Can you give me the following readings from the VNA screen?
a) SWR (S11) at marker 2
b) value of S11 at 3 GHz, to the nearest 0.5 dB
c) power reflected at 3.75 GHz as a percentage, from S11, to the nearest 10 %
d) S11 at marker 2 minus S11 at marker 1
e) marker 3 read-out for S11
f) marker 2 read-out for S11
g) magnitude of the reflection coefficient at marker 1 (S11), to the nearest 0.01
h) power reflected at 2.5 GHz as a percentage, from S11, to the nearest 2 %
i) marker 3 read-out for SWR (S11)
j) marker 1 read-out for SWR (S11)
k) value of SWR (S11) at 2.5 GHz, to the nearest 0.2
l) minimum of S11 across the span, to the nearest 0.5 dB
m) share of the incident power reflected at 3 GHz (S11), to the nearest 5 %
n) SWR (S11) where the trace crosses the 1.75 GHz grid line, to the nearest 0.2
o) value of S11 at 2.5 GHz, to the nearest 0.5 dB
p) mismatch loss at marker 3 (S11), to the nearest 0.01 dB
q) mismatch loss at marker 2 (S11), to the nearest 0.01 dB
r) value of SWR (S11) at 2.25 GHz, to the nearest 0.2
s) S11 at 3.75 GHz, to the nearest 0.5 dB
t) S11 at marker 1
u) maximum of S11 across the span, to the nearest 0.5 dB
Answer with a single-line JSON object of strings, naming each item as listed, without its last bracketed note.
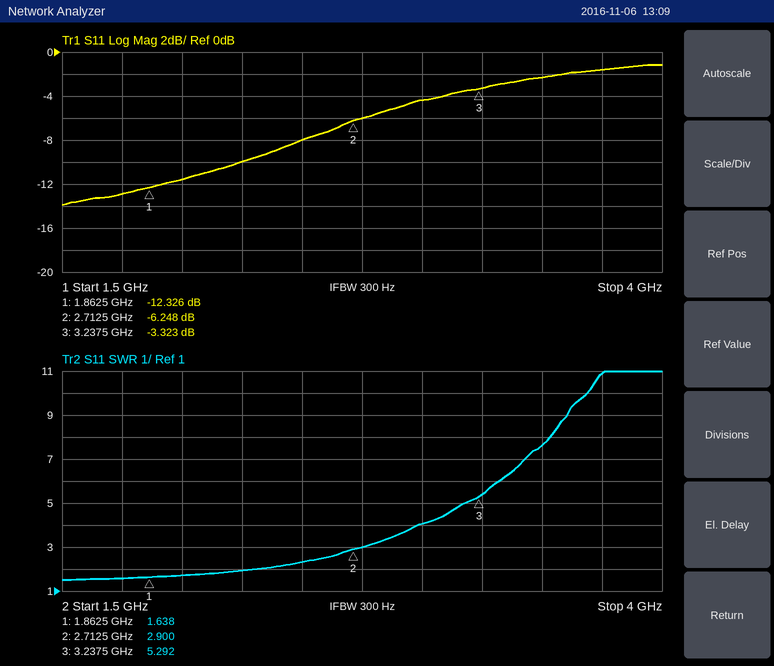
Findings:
{"SWR (S11) at marker 2": "2.900", "value of S11 at 3 GHz, to the nearest 0.5 dB": "-4.5 dB", "power reflected at 3.75 GHz as a percentage, from S11, to the nearest 10 %": "70 %", "S11 at marker 2 minus S11 at marker 1": "6.078 dB", "marker 3 read-out for S11": "-3.323 dB", "marker 2 read-out for S11": "-6.248 dB", "magnitude of the reflection coefficient at marker 1 (S11), to the nearest 0.01": "0.24", "power reflected at 2.5 GHz as a percentage, from S11, to the nearest 2 %": "16 %", "marker 3 read-out for SWR": "5.292", "marker 1 read-out for SWR": "1.638", "value of SWR (S11) at 2.5 GHz, to the nearest 0.2": "2.4", "minimum of S11 across the span, to the nearest 0.5 dB": "-14.0 dB", "share of the incident power reflected at 3 GHz (S11), to the nearest 5 %": "35 %", "SWR (S11) where the trace crosses the 1.75 GHz grid line, to the nearest 0.2": "1.6", "value of S11 at 2.5 GHz, to the nearest 0.5 dB": "-8.0 dB", "mismatch loss at marker 3 (S11), to the nearest 0.01 dB": "2.72 dB", "mismatch loss at marker 2 (S11), to the nearest 0.01 dB": "1.18 dB", "value of SWR (S11) at 2.25 GHz, to the nearest 0.2": "2.0", "S11 at 3.75 GHz, to the nearest 0.5 dB": "-1.5 dB", "S11 at marker 1": "-12.326 dB", "maximum of S11 across the span, to the nearest 0.5 dB": "-1.0 dB"}
